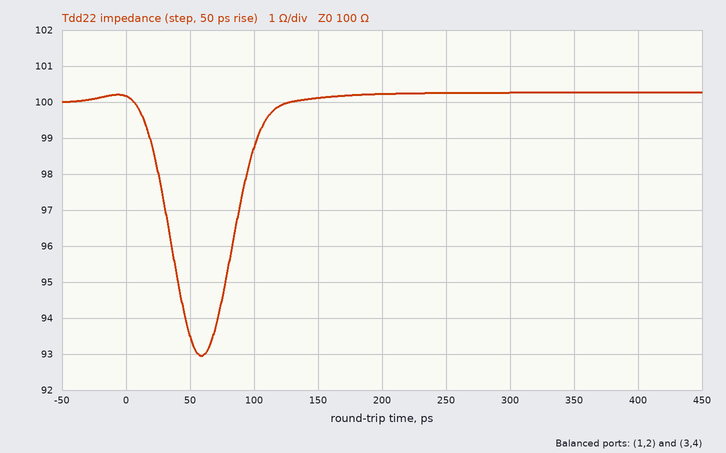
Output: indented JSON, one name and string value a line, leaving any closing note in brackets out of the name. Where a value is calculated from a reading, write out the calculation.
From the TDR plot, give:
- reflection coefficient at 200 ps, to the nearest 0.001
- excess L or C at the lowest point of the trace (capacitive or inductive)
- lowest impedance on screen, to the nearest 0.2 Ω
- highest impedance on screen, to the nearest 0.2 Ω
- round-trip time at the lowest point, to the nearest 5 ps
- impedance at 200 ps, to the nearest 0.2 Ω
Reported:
{
  "reflection coefficient at 200 ps, to the nearest 0.001": "(100.2 − 100)/(100.2 + 100) ≈ +0.001",
  "excess L or C at the lowest point of the trace": "capacitive",
  "lowest impedance on screen, to the nearest 0.2 Ω": "93.0 Ω",
  "highest impedance on screen, to the nearest 0.2 Ω": "100.2 Ω",
  "round-trip time at the lowest point, to the nearest 5 ps": "60 ps",
  "impedance at 200 ps, to the nearest 0.2 Ω": "100.2 Ω"
}
